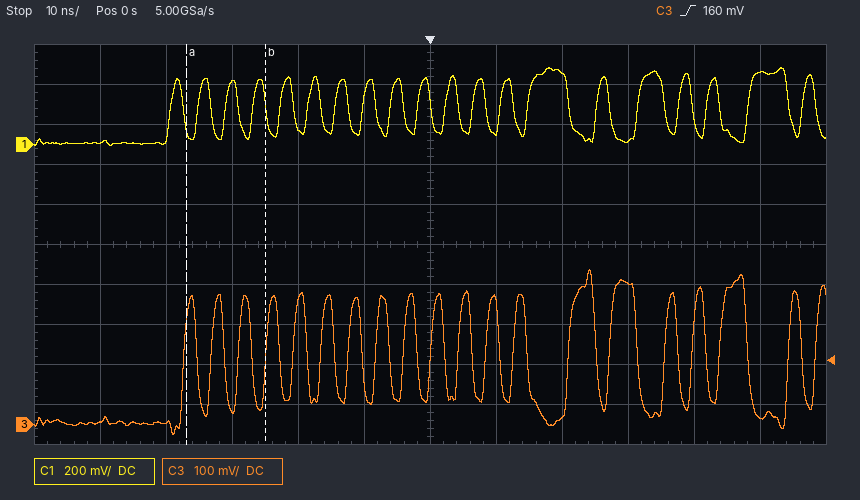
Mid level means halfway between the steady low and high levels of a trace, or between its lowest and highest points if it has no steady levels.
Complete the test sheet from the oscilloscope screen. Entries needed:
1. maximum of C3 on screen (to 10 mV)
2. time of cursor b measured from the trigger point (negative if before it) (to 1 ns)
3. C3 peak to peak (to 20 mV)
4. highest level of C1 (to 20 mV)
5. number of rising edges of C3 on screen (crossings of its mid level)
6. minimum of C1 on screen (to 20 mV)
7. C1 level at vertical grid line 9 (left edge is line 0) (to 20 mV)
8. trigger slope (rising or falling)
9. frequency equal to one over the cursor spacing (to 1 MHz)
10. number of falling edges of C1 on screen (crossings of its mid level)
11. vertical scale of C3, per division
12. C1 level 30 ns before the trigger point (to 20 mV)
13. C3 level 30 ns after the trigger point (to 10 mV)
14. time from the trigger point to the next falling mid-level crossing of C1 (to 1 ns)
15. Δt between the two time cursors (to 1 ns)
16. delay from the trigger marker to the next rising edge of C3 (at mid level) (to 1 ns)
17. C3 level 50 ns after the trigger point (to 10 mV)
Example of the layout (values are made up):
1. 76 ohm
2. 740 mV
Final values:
1. 390 mV
2. -25 ns
3. 420 mV
4. 380 mV
5. 20
6. 0 mV
7. 20 mV
8. rising
9. 83 MHz
10. 20
11. 100 mV
12. 300 mV
13. 350 mV
14. 4 ns
15. 12 ns
16. 4 ns
17. 20 mV
